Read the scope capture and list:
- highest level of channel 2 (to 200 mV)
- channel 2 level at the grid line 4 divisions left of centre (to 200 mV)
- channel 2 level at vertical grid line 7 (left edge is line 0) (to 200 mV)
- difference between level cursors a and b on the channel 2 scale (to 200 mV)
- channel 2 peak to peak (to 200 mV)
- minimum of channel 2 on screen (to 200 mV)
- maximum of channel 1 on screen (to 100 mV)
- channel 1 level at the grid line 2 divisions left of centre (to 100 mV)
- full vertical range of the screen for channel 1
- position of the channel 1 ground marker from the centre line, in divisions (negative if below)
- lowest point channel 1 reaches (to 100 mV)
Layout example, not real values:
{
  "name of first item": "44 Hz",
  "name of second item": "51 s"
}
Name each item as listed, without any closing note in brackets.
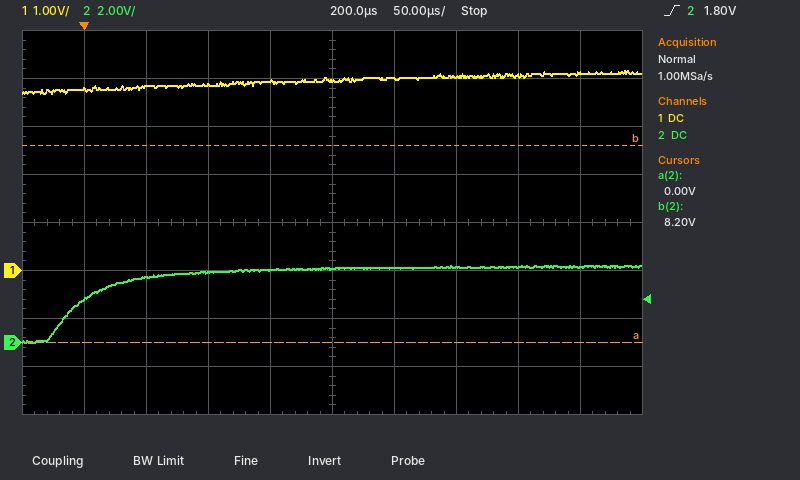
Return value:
{
  "highest level of channel 2": "3.2 V",
  "channel 2 level at the grid line 4 divisions left of centre": "1.8 V",
  "channel 2 level at vertical grid line 7 (left edge is line 0)": "3.2 V",
  "difference between level cursors a and b on the channel 2 scale": "8.2 V",
  "channel 2 peak to peak": "3.2 V",
  "minimum of channel 2 on screen": "0.0 V",
  "maximum of channel 1 on screen": "4.2 V",
  "channel 1 level at the grid line 2 divisions left of centre": "3.9 V",
  "full vertical range of the screen for channel 1": "8 V",
  "position of the channel 1 ground marker from the centre line, in divisions": "-1.0 div",
  "lowest point channel 1 reaches": "3.7 V"
}
